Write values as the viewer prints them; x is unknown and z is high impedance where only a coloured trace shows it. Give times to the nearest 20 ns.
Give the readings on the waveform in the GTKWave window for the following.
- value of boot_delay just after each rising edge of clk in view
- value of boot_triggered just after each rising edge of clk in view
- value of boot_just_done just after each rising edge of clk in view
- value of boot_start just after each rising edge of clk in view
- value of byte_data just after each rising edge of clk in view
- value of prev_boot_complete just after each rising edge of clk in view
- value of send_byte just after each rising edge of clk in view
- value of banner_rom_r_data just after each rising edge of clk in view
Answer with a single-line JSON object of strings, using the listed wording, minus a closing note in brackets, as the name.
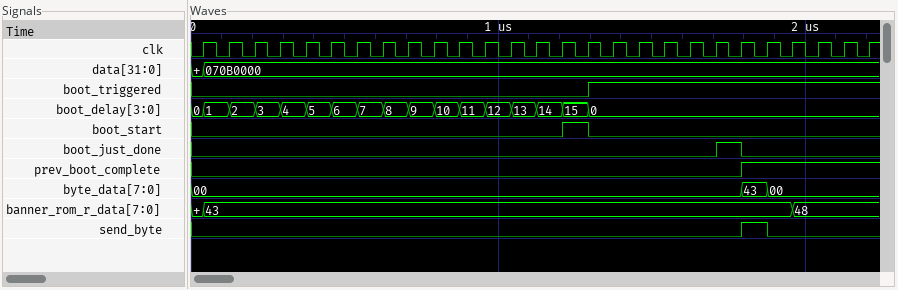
{"value of boot_delay just after each rising edge of clk in view": "1, 2, 3, 4, 5, 6, 7, 8, 9, 10, 11, 12, 13, 14, 15, 0, 0, 0, 0, 0, 0, 0, 0, 0, 0, 0, 0", "value of boot_triggered just after each rising edge of clk in view": "0 0 0 0 0 0 0 0 0 0 0 0 0 0 0 1 1 1 1 1 1 1 1 1 1 1 1", "value of boot_just_done just after each rising edge of clk in view": "0 0 0 0 0 0 0 0 0 0 0 0 0 0 0 0 0 0 0 0 1 0 0 0 0 0 0", "value of boot_start just after each rising edge of clk in view": "0 0 0 0 0 0 0 0 0 0 0 0 0 0 1 0 0 0 0 0 0 0 0 0 0 0 0", "value of byte_data just after each rising edge of clk in view": "00, 00, 00, 00, 00, 00, 00, 00, 00, 00, 00, 00, 00, 00, 00, 00, 00, 00, 00, 00, 00, 43, 00, 00, 00, 00, 00", "value of prev_boot_complete just after each rising edge of clk in view": "0 0 0 0 0 0 0 0 0 0 0 0 0 0 0 0 0 0 0 0 0 1 1 1 1 1 1", "value of send_byte just after each rising edge of clk in view": "0 0 0 0 0 0 0 0 0 0 0 0 0 0 0 0 0 0 0 0 0 1 0 0 0 0 0", "value of banner_rom_r_data just after each rising edge of clk in view": "43, 43, 43, 43, 43, 43, 43, 43, 43, 43, 43, 43, 43, 43, 43, 43, 43, 43, 43, 43, 43, 43, 43, 48, 48, 48, 48"}
